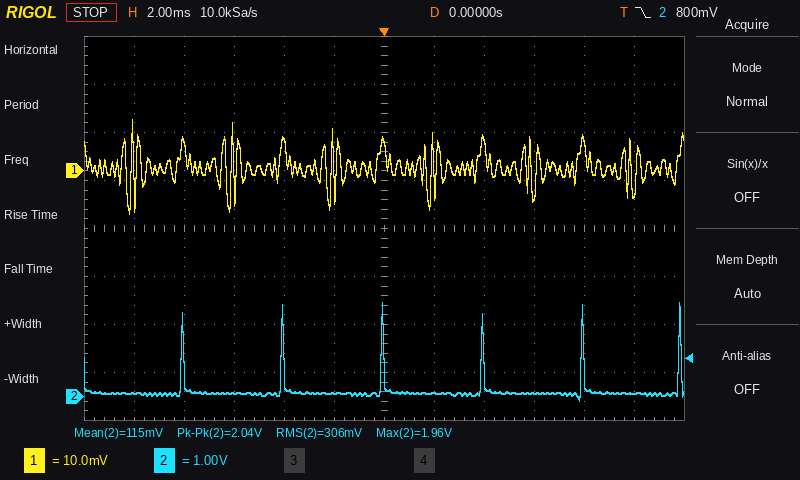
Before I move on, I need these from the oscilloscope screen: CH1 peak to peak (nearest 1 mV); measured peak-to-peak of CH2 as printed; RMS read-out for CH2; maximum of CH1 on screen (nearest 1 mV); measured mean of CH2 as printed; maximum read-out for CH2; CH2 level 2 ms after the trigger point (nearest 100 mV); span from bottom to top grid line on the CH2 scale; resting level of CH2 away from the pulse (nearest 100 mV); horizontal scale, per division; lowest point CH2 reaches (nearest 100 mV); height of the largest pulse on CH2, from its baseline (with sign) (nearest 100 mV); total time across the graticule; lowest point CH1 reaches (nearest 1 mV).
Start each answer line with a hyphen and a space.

- 20 mV
- 2.04 V
- 306 mV
- 11 mV
- 115 mV
- 1.96 V
- 100 mV
- 8 V
- 100 mV
- 2 ms
- -100 mV
- +1.9 V
- 24 ms
- -9 mV
